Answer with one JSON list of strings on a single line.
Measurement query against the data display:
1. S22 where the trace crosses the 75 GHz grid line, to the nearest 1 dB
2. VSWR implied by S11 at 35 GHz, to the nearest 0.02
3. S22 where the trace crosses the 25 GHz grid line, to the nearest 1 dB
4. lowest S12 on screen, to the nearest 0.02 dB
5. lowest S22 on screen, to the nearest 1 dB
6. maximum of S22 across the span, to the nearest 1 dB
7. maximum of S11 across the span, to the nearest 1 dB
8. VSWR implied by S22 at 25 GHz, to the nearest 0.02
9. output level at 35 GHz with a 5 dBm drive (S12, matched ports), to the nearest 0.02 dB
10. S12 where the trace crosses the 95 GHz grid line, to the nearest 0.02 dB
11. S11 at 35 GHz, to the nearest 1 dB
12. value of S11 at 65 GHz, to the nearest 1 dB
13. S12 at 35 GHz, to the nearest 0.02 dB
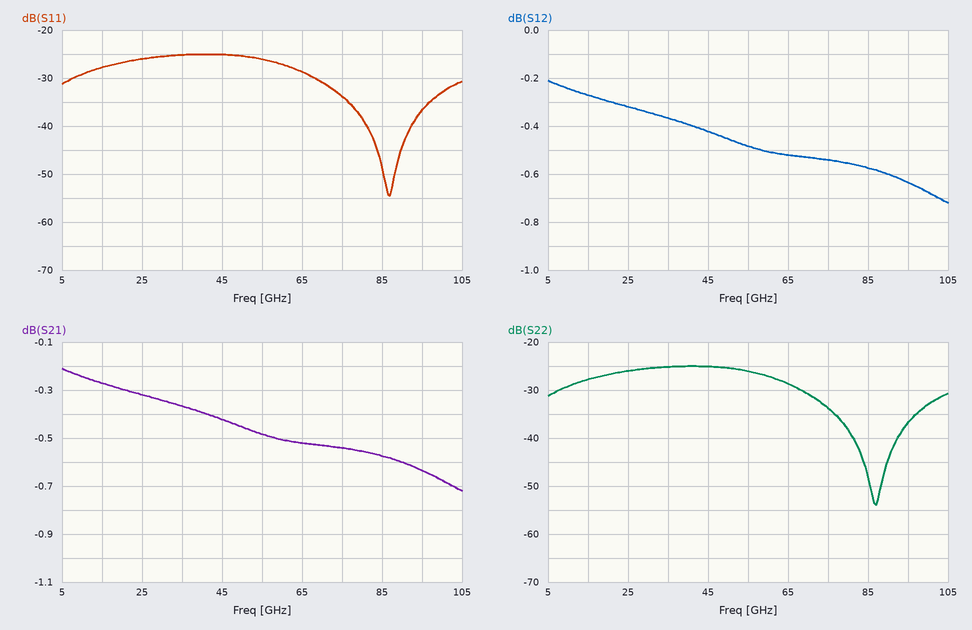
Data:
["-34 dB", "1.12", "-26 dB", "-0.72 dB", "-54 dB", "-25 dB", "-25 dB", "1.10", "4.64 dBm", "-0.64 dB", "-25 dB", "-29 dB", "-0.36 dB"]
